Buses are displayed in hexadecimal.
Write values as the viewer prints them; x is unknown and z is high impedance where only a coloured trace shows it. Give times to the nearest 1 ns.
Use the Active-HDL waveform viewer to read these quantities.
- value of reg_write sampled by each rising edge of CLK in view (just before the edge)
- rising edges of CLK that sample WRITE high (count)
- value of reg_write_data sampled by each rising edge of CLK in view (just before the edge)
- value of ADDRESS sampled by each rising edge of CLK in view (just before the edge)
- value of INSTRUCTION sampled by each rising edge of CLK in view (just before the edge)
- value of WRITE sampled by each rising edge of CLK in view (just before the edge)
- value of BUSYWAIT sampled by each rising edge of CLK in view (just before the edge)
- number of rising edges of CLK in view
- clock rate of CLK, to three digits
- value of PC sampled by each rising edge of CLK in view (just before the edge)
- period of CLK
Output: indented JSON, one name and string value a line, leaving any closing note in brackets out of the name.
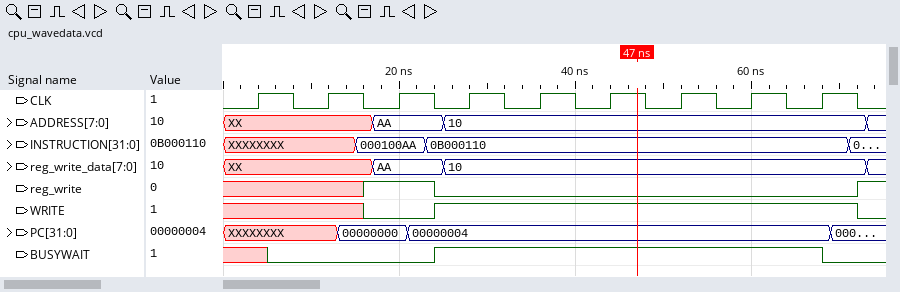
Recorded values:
{
  "value of reg_write sampled by each rising edge of CLK in view": "x x 1 0 0 0 0 0 0",
  "rising edges of CLK that sample WRITE high": "6",
  "value of reg_write_data sampled by each rising edge of CLK in view": "XX, XX, AA, 10, 10, 10, 10, 10, 10",
  "value of ADDRESS sampled by each rising edge of CLK in view": "XX, XX, AA, 10, 10, 10, 10, 10, 10",
  "value of INSTRUCTION sampled by each rising edge of CLK in view": "XXXXXXXX, XXXXXXXX, 000100AA, 0B000110, 0B000110, 0B000110, 0B000110, 0B000110, 0B000110",
  "value of WRITE sampled by each rising edge of CLK in view": "x x 0 1 1 1 1 1 1",
  "value of BUSYWAIT sampled by each rising edge of CLK in view": "x 0 0 1 1 1 1 1 1",
  "number of rising edges of CLK in view": "9",
  "clock rate of CLK, to three digits": "125 MHz",
  "value of PC sampled by each rising edge of CLK in view": "XXXXXXXX, XXXXXXXX, 00000000, 00000004, 00000004, 00000004, 00000004, 00000004, 00000004",
  "period of CLK": "8 ns"
}
